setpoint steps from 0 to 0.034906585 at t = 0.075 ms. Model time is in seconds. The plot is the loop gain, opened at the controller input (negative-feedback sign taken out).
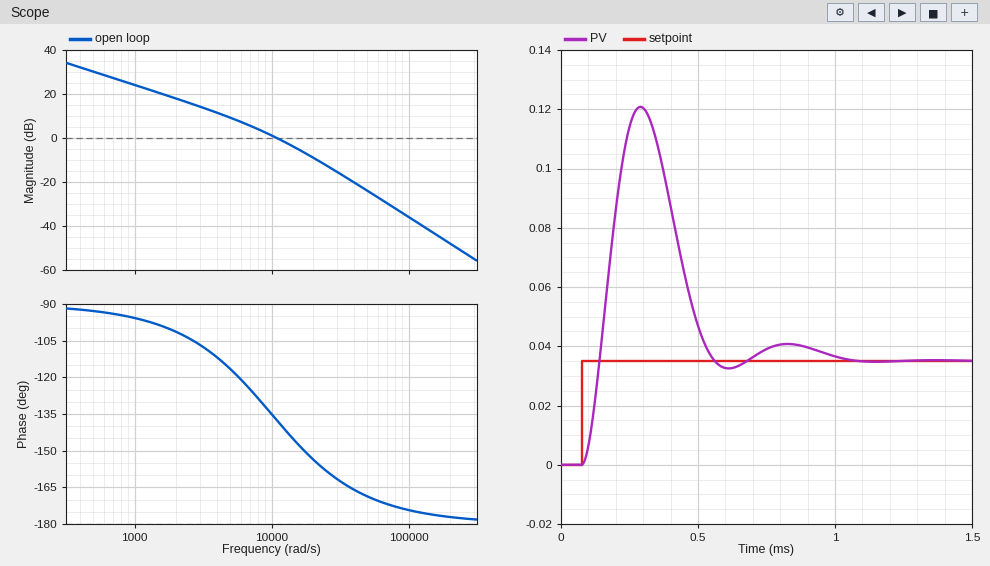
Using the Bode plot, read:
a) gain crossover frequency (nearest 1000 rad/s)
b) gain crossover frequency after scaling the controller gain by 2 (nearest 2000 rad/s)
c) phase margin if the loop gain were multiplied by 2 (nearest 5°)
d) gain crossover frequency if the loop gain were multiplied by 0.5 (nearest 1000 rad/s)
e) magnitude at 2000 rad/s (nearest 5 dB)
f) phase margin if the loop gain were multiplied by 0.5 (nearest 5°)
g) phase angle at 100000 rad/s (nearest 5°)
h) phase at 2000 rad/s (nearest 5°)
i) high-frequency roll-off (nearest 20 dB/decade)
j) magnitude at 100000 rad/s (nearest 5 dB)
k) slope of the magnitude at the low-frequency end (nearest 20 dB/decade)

11000 rad/s
16000 rad/s
30°
7000 rad/s
20 dB
55°
-175°
-100°
-40 dB/decade
-35 dB
-20 dB/decade
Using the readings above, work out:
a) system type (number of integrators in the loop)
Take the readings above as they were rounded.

1
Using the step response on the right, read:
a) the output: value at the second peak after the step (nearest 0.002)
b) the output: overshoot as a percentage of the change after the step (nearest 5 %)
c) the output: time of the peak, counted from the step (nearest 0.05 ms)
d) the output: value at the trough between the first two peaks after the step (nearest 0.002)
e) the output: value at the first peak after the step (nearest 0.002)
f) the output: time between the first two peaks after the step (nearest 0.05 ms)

0.040
245 %
0.20 ms
0.032
0.120
0.55 ms
